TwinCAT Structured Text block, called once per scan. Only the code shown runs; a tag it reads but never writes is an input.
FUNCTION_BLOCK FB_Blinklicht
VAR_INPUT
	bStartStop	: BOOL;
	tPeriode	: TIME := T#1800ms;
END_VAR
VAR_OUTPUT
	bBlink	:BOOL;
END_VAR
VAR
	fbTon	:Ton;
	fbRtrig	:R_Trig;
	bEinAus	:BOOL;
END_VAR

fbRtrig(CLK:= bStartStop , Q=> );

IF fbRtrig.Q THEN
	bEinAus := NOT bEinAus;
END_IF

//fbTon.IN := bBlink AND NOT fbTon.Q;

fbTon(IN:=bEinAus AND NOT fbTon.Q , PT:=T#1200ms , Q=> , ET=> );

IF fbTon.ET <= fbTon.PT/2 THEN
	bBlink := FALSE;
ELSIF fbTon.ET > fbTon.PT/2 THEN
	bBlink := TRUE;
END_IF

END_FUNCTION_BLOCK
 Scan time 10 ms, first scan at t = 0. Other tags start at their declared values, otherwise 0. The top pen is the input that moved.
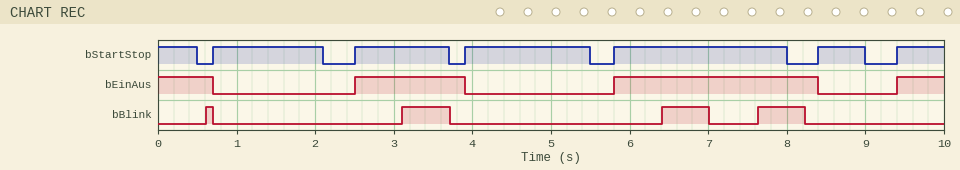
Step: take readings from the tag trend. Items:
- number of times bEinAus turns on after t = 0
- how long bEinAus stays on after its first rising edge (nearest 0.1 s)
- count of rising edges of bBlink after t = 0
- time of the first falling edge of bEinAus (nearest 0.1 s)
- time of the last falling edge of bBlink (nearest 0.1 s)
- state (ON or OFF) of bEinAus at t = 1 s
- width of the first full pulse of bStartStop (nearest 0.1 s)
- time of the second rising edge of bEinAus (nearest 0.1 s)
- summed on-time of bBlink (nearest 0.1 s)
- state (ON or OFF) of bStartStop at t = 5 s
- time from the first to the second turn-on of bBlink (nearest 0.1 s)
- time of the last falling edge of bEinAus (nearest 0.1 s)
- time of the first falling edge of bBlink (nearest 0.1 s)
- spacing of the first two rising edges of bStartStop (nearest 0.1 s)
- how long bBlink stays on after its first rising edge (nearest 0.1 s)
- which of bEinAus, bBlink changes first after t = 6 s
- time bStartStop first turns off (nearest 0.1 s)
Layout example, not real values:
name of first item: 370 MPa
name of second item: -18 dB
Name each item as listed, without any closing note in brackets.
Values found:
number of times bEinAus turns on after t = 0: 3
how long bEinAus stays on after its first rising edge: 1.4 s
count of rising edges of bBlink after t = 0: 4
time of the first falling edge of bEinAus: 0.7 s
time of the last falling edge of bBlink: 8.2 s
state (ON or OFF) of bEinAus at t = 1 s: OFF
width of the first full pulse of bStartStop: 1.4 s
time of the second rising edge of bEinAus: 5.8 s
summed on-time of bBlink: 1.9 s
state (ON or OFF) of bStartStop at t = 5 s: ON
time from the first to the second turn-on of bBlink: 2.5 s
time of the last falling edge of bEinAus: 8.4 s
time of the first falling edge of bBlink: 0.7 s
spacing of the first two rising edges of bStartStop: 1.8 s
how long bBlink stays on after its first rising edge: 0.1 s
which of bEinAus, bBlink changes first after t = 6 s: bBlink
time bStartStop first turns off: 0.5 s
